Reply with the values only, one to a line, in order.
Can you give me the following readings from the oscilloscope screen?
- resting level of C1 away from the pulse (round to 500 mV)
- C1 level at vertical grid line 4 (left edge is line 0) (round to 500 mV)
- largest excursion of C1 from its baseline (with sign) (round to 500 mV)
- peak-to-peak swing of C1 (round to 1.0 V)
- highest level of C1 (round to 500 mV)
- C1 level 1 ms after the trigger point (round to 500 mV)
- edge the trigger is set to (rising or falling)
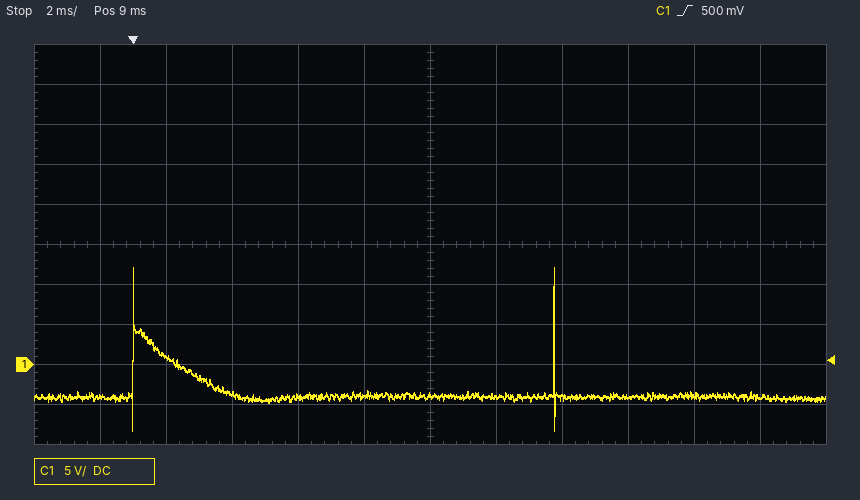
-4.0 V
-4.0 V
+16.0 V
20.0 V
12.0 V
1.0 V
rising
